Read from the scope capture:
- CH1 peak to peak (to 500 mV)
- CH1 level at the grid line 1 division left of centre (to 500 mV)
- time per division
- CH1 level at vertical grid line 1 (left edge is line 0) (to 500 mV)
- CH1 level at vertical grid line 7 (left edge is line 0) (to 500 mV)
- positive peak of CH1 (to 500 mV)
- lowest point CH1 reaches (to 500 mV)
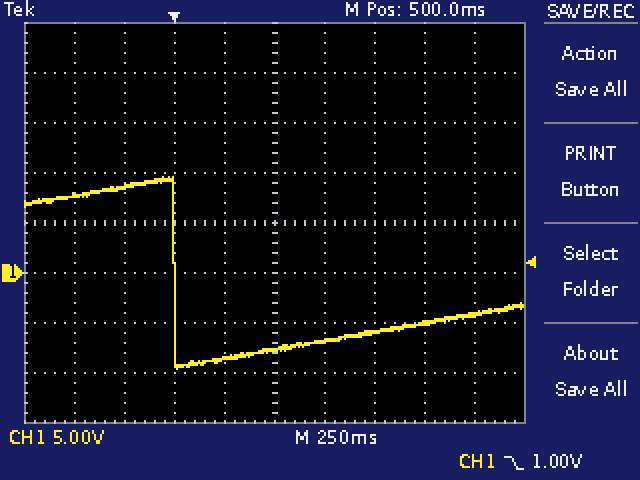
19.0 V
-8.5 V
250 ms
8.0 V
-6.0 V
9.5 V
-9.5 V
